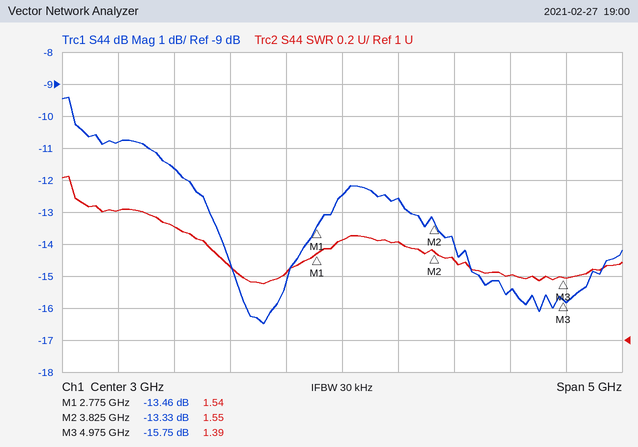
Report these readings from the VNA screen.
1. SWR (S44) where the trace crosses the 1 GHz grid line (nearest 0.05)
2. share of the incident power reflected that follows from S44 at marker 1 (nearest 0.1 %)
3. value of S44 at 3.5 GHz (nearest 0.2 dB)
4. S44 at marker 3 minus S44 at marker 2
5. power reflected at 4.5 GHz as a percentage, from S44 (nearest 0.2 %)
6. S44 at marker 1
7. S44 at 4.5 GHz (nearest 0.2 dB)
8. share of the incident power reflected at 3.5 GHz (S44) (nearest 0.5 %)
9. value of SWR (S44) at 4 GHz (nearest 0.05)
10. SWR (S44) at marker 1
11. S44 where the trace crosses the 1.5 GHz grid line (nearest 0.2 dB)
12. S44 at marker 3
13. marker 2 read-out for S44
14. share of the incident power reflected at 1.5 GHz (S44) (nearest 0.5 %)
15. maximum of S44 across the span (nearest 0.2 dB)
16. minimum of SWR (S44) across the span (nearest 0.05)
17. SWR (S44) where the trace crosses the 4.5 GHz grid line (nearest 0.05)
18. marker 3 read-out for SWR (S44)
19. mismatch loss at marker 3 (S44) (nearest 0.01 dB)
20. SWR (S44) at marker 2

1.80
4.5 %
-12.6 dB
-2.42 dB
2.8 %
-13.46 dB
-15.4 dB
5.5 %
1.50
1.54
-11.6 dB
-15.75 dB
-13.33 dB
7.0 %
-9.4 dB
1.35
1.40
1.39
0.12 dB
1.55
